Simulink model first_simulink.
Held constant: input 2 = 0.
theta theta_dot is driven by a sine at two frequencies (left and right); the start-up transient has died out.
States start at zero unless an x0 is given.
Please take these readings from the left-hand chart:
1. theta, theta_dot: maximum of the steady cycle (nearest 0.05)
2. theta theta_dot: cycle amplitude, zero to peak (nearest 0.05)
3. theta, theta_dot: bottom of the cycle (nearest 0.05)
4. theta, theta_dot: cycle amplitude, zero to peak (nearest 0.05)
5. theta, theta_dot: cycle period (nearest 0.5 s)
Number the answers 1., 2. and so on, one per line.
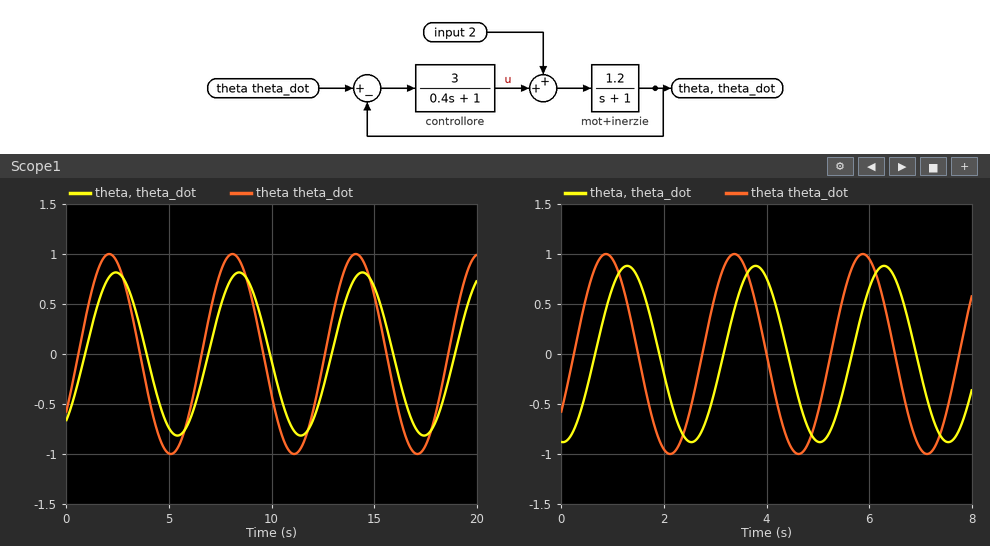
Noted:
1. 0.80
2. 1.00
3. -0.80
4. 0.80
5. 6.0 s
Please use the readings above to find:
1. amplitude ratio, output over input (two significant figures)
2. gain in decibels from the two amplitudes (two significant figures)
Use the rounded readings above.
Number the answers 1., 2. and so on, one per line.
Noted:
1. 0.80
2. -1.9 dB
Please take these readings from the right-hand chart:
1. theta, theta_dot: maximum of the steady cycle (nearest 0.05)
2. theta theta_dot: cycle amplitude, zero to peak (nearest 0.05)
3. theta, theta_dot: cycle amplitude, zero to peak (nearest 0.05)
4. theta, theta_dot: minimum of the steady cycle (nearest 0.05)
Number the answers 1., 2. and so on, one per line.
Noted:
1. 0.90
2. 1.00
3. 0.90
4. -0.90
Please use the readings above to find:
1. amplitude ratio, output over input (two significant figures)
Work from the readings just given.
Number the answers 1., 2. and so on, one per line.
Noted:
1. 0.90
